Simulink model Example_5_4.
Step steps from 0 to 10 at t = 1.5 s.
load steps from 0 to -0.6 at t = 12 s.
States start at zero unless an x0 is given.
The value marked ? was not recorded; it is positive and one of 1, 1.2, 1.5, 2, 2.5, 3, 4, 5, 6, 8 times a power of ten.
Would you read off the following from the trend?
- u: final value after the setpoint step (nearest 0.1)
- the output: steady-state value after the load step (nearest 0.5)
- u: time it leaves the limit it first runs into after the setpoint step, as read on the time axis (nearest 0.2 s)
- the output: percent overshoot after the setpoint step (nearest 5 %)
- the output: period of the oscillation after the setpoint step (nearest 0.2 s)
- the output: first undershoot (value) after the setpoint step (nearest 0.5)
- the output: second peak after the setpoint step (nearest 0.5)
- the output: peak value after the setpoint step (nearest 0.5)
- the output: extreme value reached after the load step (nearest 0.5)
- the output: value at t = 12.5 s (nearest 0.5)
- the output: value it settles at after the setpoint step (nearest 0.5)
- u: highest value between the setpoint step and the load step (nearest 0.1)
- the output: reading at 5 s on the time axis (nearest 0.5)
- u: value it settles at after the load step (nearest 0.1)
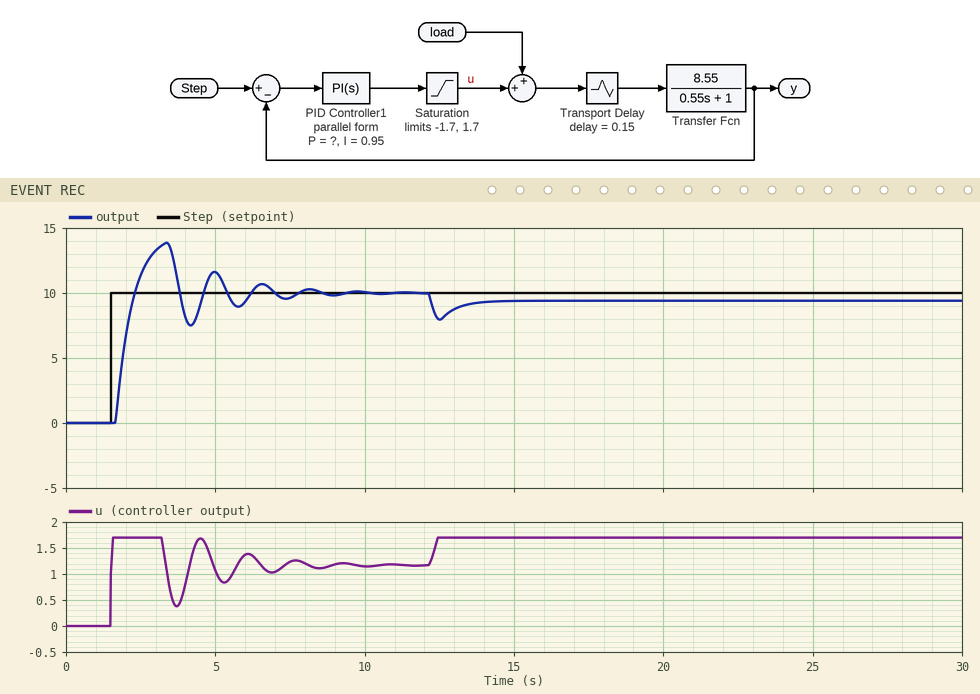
1.2
9.5
3.2 s
40 %
1.6 s
7.5
11.5
14.0
8.0
8.0
10.0
1.7
11.5
1.7
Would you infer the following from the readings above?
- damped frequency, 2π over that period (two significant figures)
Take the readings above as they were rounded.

3.9 rad/s
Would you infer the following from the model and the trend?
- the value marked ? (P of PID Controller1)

0.1
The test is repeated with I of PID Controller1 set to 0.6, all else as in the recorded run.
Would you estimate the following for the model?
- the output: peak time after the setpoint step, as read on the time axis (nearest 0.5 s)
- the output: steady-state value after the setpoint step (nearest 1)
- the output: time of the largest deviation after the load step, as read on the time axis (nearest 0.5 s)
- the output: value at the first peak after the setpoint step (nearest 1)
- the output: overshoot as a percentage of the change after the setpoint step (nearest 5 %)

3.0 s
10
12.5 s
13
35 %
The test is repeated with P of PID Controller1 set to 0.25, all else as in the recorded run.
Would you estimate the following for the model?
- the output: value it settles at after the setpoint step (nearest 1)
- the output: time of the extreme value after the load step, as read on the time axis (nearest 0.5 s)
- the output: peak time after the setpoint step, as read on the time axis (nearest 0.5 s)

10
12.5 s
3.0 s
